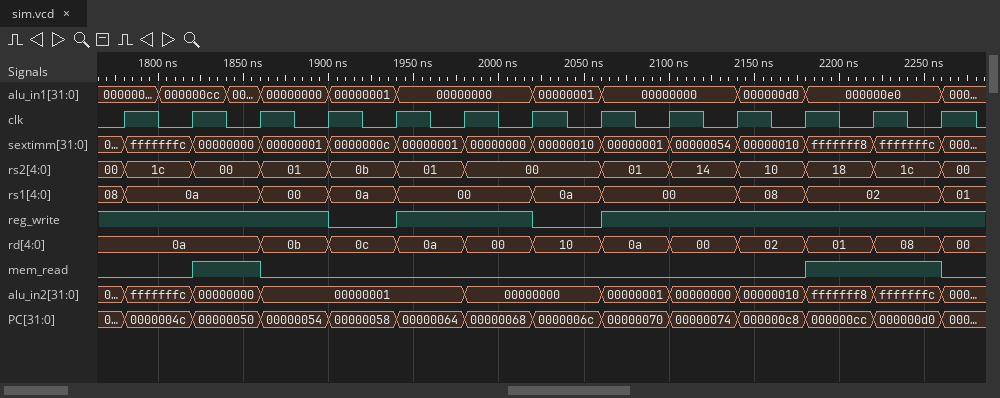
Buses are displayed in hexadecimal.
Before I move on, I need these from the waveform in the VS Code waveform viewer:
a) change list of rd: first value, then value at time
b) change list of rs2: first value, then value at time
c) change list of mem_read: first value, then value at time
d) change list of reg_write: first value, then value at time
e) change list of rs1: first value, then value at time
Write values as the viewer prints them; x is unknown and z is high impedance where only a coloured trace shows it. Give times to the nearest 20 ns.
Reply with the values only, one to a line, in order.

0a, 0b at 1860 ns, 0c at 1900 ns, 0a at 1940 ns, 00 at 1980 ns, 10 at 2020 ns, 0a at 2060 ns, 00 at 2100 ns, 02 at 2140 ns, 01 at 2180 ns, 08 at 2220 ns, 00 at 2260 ns
00, 1c at 1780 ns, 00 at 1820 ns, 01 at 1860 ns, 0b at 1900 ns, 01 at 1940 ns, 00 at 1980 ns, 01 at 2060 ns, 14 at 2100 ns, 10 at 2140 ns, 18 at 2180 ns, 1c at 2220 ns, 00 at 2260 ns
0, 1 at 1820 ns, 0 at 1860 ns, 1 at 2180 ns, 0 at 2260 ns
1, 0 at 1900 ns, 1 at 1940 ns, 0 at 2020 ns, 1 at 2060 ns
08, 0a at 1780 ns, 00 at 1860 ns, 0a at 1900 ns, 00 at 1940 ns, 0a at 2020 ns, 00 at 2060 ns, 08 at 2140 ns, 02 at 2180 ns, 01 at 2260 ns
